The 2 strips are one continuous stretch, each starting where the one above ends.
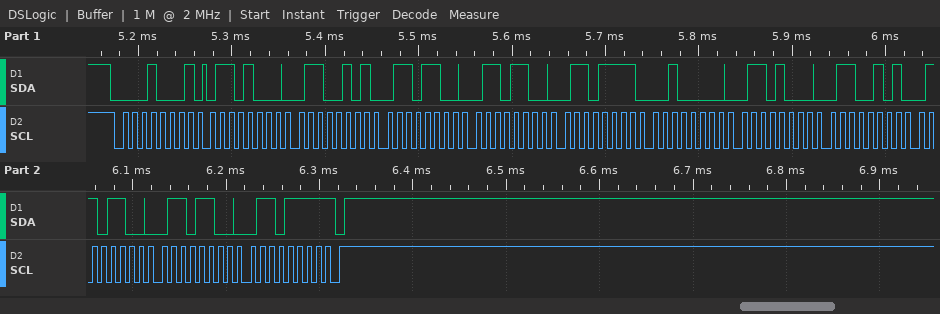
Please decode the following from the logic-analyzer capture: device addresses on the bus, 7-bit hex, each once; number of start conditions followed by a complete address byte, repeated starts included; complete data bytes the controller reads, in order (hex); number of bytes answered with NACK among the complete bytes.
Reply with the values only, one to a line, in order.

0x08
1
68 65 6C 6C 6F 20 68 65 6C 6C 6F
1
